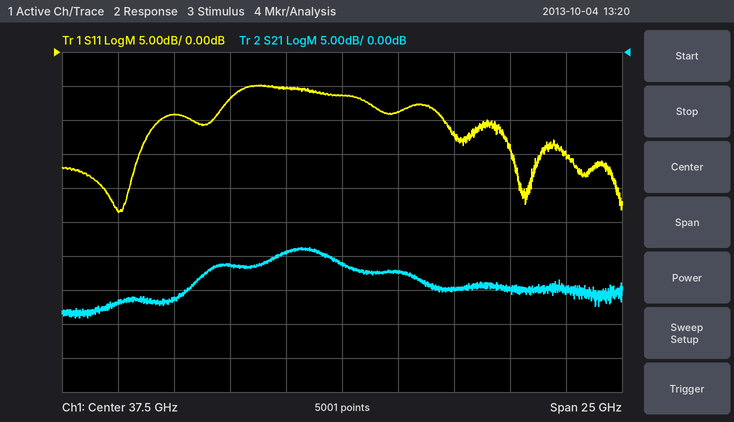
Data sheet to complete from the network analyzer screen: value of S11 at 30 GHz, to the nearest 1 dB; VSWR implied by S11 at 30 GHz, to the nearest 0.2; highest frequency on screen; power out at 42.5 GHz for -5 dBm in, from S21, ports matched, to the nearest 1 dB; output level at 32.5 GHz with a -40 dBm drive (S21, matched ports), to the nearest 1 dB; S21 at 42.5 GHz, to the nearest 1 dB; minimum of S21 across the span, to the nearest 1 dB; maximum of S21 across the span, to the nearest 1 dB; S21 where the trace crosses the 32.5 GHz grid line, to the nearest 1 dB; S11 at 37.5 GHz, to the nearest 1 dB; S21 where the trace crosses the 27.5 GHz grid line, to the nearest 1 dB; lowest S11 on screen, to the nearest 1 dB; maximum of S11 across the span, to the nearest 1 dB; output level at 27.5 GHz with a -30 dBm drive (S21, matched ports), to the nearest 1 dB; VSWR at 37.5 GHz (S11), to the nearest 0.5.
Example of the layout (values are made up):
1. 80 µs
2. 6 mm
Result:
1. -9 dB
2. 2.0
3. 50 GHz
4. -40 dBm
5. -71 dBm
6. -35 dB
7. -39 dB
8. -29 dB
9. -31 dB
10. -6 dB
11. -37 dB
12. -24 dB
13. -5 dB
14. -67 dBm
15. 3.0
